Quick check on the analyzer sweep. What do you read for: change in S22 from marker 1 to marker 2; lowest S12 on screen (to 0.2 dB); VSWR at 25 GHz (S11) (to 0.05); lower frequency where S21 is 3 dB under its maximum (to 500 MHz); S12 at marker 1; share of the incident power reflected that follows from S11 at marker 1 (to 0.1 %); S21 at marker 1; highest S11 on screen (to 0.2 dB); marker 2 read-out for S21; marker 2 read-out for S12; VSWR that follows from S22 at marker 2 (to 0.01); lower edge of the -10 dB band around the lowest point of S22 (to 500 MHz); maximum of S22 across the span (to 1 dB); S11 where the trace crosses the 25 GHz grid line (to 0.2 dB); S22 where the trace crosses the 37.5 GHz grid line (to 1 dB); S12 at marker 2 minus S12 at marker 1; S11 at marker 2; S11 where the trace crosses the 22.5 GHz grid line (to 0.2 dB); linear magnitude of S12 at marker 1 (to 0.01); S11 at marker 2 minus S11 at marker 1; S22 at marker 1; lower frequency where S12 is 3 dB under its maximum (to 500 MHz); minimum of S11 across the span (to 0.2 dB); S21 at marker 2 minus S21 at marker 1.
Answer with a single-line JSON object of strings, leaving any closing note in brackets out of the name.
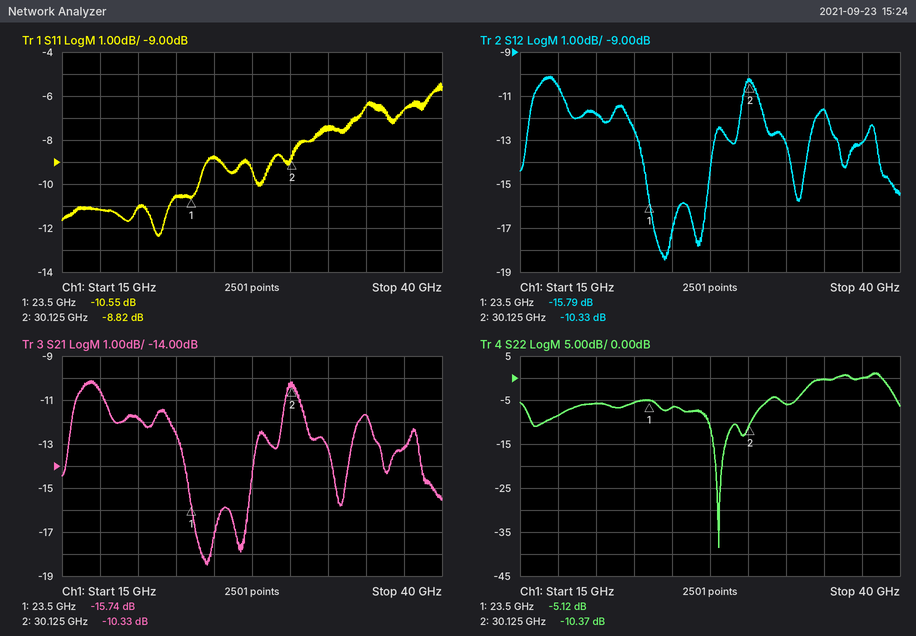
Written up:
{"change in S22 from marker 1 to marker 2": "-5.25 dB", "lowest S12 on screen": "-18.4 dB", "VSWR at 25 GHz (S11)": "2.15", "lower frequency where S21 is 3 dB under its maximum": "15.5 GHz", "S12 at marker 1": "-15.79 dB", "share of the incident power reflected that follows from S11 at marker 1": "8.8 %", "S21 at marker 1": "-15.74 dB", "highest S11 on screen": "-5.4 dB", "marker 2 read-out for S21": "-10.33 dB", "marker 2 read-out for S12": "-10.33 dB", "VSWR that follows from S22 at marker 2": "1.87", "lower edge of the -10 dB band around the lowest point of S22": "27.5 GHz", "maximum of S22 across the span": "1 dB", "S11 where the trace crosses the 25 GHz grid line": "-8.8 dB", "S22 where the trace crosses the 37.5 GHz grid line": "0 dB", "S12 at marker 2 minus S12 at marker 1": "5.46 dB", "S11 at marker 2": "-8.82 dB", "S11 where the trace crosses the 22.5 GHz grid line": "-10.6 dB", "linear magnitude of S12 at marker 1": "0.16", "S11 at marker 2 minus S11 at marker 1": "1.73 dB", "S22 at marker 1": "-5.12 dB", "lower frequency where S12 is 3 dB under its maximum": "15.5 GHz", "minimum of S11 across the span": "-12.4 dB", "S21 at marker 2 minus S21 at marker 1": "5.41 dB"}
